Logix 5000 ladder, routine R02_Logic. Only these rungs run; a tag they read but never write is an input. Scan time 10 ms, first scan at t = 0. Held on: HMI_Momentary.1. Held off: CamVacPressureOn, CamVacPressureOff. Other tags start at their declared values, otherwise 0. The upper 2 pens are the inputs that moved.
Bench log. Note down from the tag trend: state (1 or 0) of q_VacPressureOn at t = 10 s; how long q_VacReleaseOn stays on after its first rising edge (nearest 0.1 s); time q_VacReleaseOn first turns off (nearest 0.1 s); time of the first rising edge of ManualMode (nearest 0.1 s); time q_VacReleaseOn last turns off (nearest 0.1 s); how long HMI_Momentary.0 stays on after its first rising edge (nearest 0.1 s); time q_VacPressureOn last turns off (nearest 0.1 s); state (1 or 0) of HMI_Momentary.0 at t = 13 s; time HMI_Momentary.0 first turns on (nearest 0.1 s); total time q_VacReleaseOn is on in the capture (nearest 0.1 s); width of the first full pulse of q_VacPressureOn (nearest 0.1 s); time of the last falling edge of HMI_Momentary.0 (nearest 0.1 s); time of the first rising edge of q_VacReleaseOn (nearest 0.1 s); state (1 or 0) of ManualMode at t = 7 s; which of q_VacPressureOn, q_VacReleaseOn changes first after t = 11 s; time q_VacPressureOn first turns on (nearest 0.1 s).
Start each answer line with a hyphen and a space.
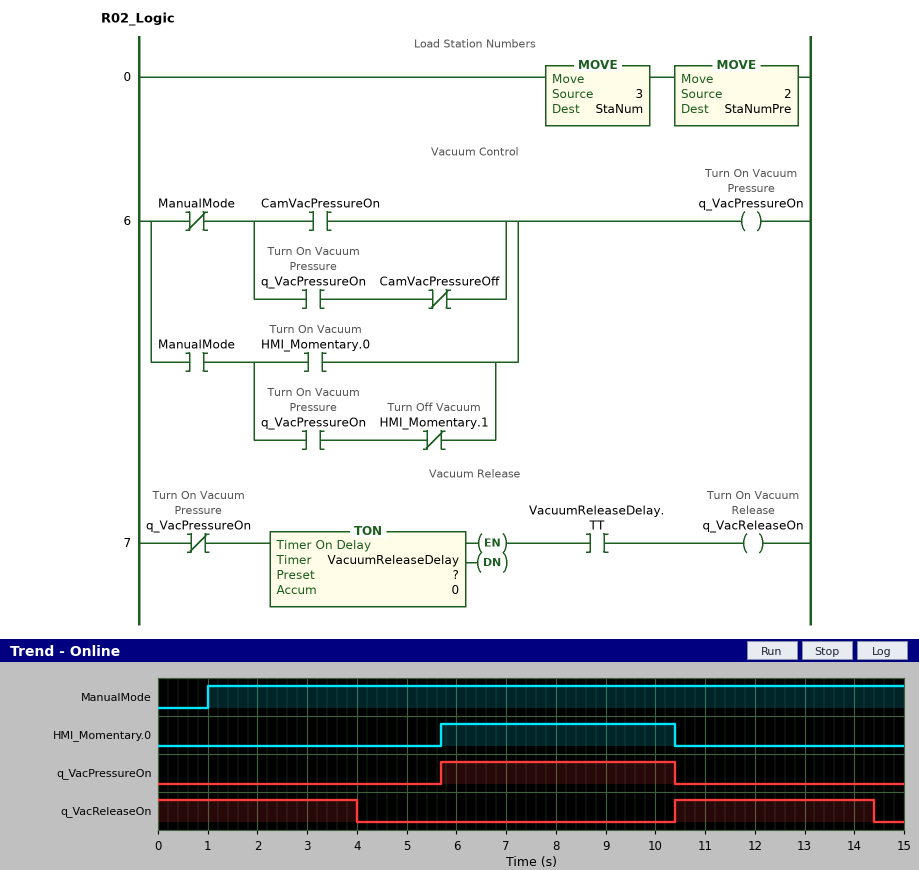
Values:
- 1
- 4.0 s
- 4.0 s
- 1.0 s
- 14.4 s
- 4.7 s
- 10.4 s
- 0
- 5.7 s
- 8.0 s
- 4.7 s
- 10.4 s
- 10.4 s
- 1
- q_VacReleaseOn
- 5.7 s
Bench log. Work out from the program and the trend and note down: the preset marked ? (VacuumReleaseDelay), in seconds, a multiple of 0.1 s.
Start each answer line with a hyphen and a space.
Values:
- 4.0 s
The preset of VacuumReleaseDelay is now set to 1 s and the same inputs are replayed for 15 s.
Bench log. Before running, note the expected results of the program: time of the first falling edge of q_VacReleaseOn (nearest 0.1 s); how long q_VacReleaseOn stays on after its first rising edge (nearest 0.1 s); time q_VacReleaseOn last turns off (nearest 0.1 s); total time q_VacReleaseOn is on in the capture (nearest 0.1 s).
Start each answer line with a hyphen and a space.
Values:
- 1.0 s
- 1.0 s
- 11.4 s
- 2.0 s
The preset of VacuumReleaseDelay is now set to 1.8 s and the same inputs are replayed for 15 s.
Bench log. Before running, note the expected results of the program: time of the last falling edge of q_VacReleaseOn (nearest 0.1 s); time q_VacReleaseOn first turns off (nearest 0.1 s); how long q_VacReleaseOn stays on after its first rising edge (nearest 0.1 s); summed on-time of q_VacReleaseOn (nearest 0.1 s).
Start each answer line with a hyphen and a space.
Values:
- 12.2 s
- 1.8 s
- 1.8 s
- 3.6 s
